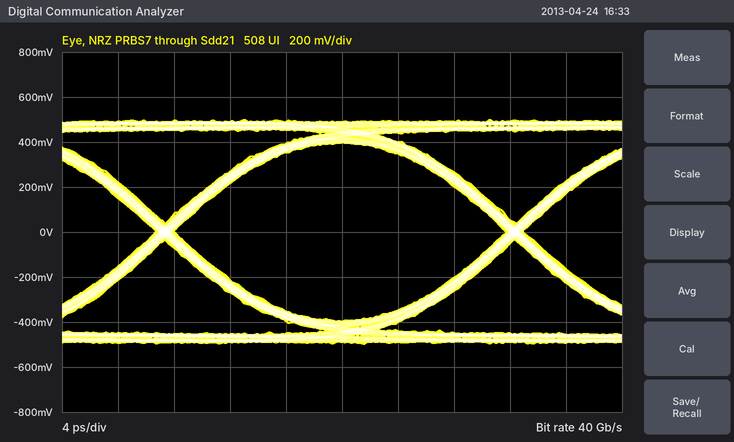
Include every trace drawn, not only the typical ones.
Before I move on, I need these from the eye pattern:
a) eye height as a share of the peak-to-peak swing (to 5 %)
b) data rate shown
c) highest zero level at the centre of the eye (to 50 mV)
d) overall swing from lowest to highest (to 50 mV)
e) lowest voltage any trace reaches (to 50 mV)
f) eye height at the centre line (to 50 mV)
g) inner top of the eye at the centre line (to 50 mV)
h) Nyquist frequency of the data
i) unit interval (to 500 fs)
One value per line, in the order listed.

80 %
40 Gb/s
-400 mV
1.00 V
-500 mV
800 mV
400 mV
20 GHz
25.0 ps
